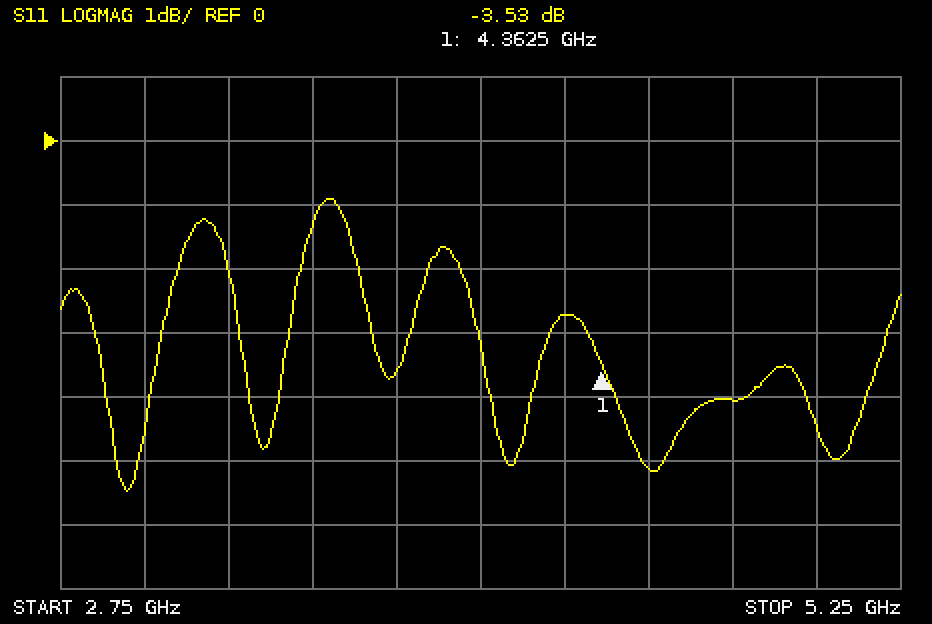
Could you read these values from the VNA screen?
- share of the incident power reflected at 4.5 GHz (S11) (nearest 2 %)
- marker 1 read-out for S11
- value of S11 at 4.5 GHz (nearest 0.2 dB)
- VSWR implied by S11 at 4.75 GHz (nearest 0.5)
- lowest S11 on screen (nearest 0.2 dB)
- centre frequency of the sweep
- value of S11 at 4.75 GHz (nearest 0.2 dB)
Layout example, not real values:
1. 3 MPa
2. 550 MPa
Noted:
1. 30 %
2. -3.53 dB
3. -5.2 dB
4. 4.5
5. -5.4 dB
6. 4 GHz
7. -4.0 dB
